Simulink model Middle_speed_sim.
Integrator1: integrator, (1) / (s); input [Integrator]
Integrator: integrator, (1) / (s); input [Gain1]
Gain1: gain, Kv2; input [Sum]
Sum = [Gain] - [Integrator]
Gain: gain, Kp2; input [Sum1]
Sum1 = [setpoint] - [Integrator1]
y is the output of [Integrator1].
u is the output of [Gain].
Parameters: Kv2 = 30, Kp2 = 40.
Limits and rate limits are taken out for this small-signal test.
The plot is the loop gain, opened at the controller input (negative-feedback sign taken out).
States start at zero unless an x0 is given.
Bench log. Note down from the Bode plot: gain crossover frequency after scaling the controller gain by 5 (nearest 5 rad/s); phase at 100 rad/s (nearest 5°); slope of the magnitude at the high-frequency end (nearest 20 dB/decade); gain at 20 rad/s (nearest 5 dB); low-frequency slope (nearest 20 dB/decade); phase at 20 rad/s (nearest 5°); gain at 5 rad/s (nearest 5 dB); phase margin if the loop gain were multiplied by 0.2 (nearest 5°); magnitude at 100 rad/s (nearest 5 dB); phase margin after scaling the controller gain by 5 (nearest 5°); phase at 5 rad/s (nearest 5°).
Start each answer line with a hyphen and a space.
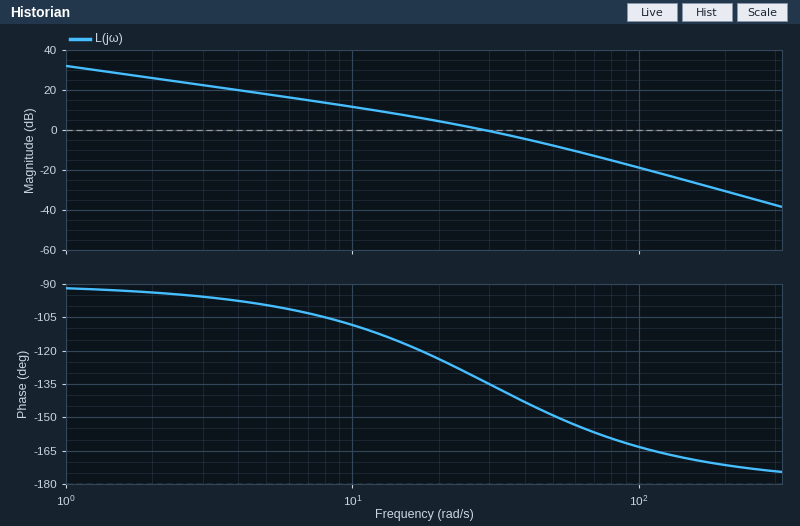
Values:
- 75 rad/s
- -165°
- -40 dB/decade
- 5 dB
- -20 dB/decade
- -125°
- 20 dB
- 75°
- -20 dB
- 20°
- -100°
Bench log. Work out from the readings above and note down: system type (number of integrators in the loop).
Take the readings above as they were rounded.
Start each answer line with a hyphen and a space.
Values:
- 1
